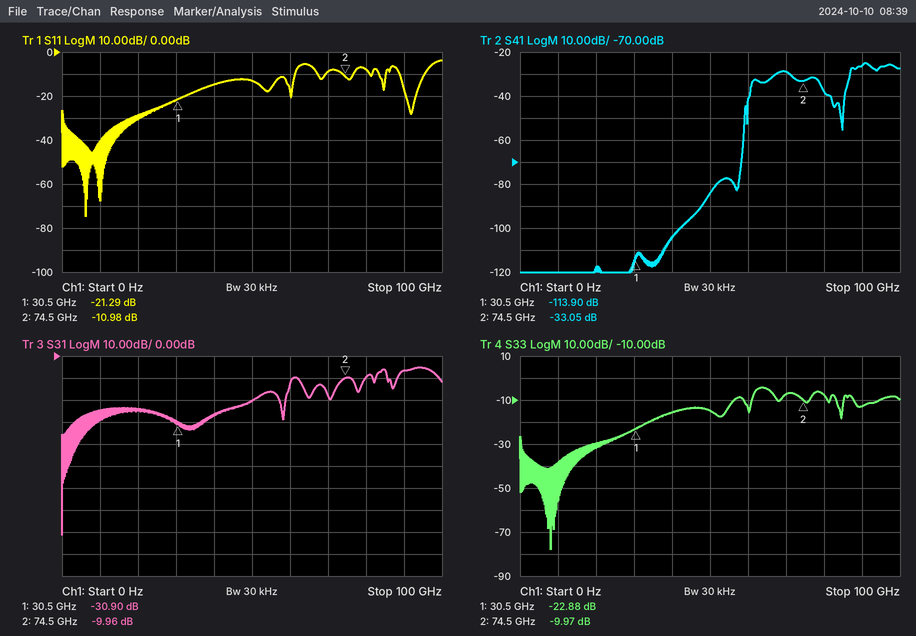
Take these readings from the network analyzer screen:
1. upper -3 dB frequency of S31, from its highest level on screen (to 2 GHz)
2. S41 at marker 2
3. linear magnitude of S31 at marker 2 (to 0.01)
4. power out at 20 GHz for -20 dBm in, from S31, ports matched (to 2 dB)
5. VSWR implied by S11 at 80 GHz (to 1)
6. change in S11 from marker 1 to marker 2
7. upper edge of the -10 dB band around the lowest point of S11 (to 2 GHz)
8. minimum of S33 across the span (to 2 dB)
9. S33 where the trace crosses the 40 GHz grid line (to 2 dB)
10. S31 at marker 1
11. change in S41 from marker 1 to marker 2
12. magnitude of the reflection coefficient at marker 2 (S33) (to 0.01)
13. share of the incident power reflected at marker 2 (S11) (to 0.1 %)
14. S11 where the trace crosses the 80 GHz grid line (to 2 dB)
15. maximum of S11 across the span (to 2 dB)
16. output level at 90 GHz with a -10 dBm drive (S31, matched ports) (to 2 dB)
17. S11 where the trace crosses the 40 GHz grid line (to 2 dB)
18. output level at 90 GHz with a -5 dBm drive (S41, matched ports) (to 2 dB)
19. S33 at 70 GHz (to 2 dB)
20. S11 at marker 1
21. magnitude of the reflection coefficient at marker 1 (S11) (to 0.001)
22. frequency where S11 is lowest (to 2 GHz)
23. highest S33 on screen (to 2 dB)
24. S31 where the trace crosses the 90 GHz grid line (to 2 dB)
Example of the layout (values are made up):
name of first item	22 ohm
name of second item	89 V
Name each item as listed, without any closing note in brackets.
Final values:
upper -3 dB frequency of S31, from its highest level on screen	98 GHz
S41 at marker 2	-33.05 dB
linear magnitude of S31 at marker 2	0.32
power out at 20 GHz for -20 dBm in, from S31, ports matched	-44 dBm
VSWR implied by S11 at 80 GHz	2
change in S11 from marker 1 to marker 2	10.31 dB
upper edge of the -10 dB band around the lowest point of S11	62 GHz
minimum of S33 across the span	-78 dB
S33 where the trace crosses the 40 GHz grid line	-16 dB
S31 at marker 1	-30.90 dB
change in S41 from marker 1 to marker 2	80.85 dB
magnitude of the reflection coefficient at marker 2 (S33)	0.32
share of the incident power reflected at marker 2 (S11)	8.0 %
S11 where the trace crosses the 80 GHz grid line	-8 dB
maximum of S11 across the span	-4 dB
output level at 90 GHz with a -10 dBm drive (S31, matched ports)	-16 dBm
S11 where the trace crosses the 40 GHz grid line	-14 dB
output level at 90 GHz with a -5 dBm drive (S41, matched ports)	-32 dBm
S33 at 70 GHz	-8 dB
S11 at marker 1	-21.29 dB
magnitude of the reflection coefficient at marker 1 (S11)	0.086
frequency where S11 is lowest	6 GHz
highest S33 on screen	-4 dB
S31 where the trace crosses the 90 GHz grid line	-6 dB
